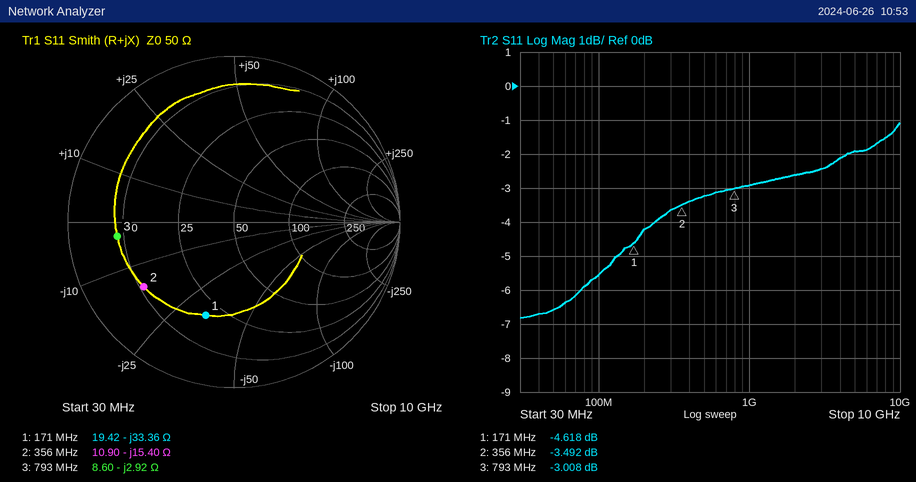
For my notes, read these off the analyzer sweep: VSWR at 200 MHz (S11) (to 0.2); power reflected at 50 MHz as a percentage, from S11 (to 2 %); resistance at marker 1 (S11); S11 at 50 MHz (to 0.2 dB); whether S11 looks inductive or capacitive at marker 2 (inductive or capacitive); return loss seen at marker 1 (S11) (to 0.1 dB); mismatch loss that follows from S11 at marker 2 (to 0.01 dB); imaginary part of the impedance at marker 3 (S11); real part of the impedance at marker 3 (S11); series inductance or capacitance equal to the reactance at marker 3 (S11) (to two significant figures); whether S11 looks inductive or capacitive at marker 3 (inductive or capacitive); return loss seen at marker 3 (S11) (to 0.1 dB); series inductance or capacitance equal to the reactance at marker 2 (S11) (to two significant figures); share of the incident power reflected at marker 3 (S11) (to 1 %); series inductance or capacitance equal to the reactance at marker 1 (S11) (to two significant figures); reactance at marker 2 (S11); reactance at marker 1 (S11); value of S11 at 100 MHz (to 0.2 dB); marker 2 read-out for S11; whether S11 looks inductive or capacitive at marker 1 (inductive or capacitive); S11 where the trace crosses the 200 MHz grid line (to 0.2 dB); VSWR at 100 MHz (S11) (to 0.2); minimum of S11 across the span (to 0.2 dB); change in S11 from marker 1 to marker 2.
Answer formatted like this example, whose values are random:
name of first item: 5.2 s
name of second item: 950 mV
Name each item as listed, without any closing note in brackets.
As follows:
VSWR at 200 MHz (S11): 4.2
power reflected at 50 MHz as a percentage, from S11: 22 %
resistance at marker 1: 19.42 Ω
S11 at 50 MHz: -6.6 dB
whether S11 looks inductive or capacitive at marker 2: capacitive
return loss seen at marker 1 (S11): 4.6 dB
mismatch loss that follows from S11 at marker 2: 2.58 dB
imaginary part of the impedance at marker 3: -2.92 Ω
real part of the impedance at marker 3: 8.60 Ω
series inductance or capacitance equal to the reactance at marker 3 (S11): 69 pF
whether S11 looks inductive or capacitive at marker 3: capacitive
return loss seen at marker 3 (S11): 3.0 dB
series inductance or capacitance equal to the reactance at marker 2 (S11): 29 pF
share of the incident power reflected at marker 3 (S11): 50 %
series inductance or capacitance equal to the reactance at marker 1 (S11): 28 pF
reactance at marker 2: -15.40 Ω
reactance at marker 1: -33.36 Ω
value of S11 at 100 MHz: -5.6 dB
marker 2 read-out for S11: -3.492 dB
whether S11 looks inductive or capacitive at marker 1: capacitive
S11 where the trace crosses the 200 MHz grid line: -4.2 dB
VSWR at 100 MHz (S11): 3.2
minimum of S11 across the span: -6.8 dB
change in S11 from marker 1 to marker 2: 1.126 dB
